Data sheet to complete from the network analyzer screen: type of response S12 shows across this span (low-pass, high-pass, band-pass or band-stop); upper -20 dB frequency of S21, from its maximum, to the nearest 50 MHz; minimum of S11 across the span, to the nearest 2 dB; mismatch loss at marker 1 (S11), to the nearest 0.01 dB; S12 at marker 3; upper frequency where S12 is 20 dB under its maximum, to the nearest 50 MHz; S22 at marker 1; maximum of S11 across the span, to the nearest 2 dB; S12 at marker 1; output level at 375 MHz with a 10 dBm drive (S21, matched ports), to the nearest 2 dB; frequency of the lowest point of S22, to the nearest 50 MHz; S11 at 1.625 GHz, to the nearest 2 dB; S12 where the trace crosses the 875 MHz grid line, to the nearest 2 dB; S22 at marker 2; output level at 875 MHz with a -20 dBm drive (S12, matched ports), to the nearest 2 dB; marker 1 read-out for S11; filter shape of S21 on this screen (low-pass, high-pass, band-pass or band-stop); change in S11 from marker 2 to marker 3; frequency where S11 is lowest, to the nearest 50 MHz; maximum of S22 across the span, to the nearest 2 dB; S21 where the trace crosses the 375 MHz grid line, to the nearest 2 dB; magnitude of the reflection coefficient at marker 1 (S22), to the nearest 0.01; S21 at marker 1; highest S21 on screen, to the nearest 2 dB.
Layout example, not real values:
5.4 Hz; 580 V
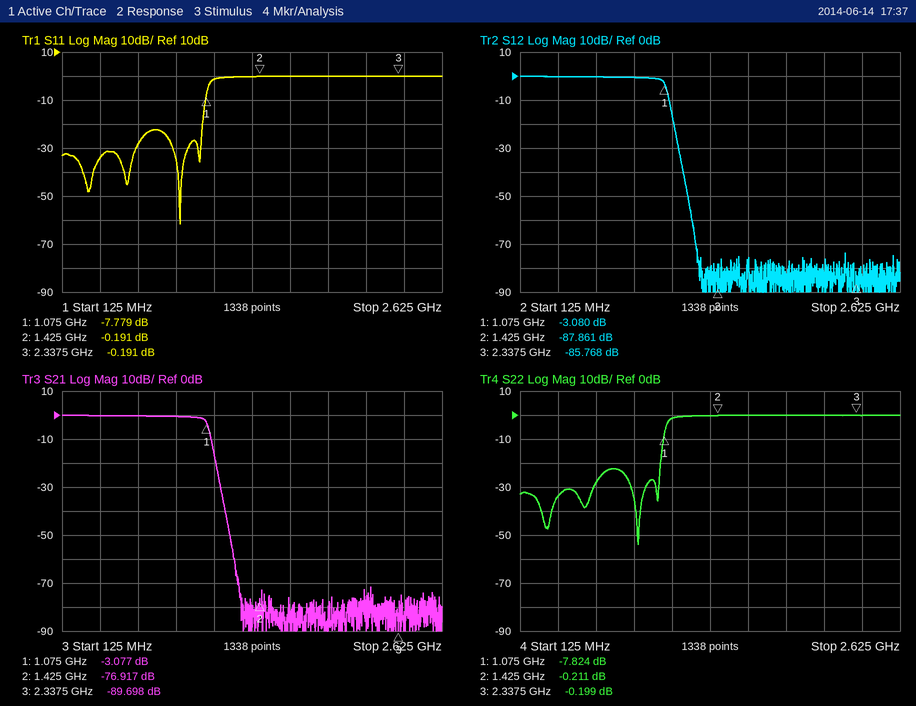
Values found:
low-pass; 1.15 GHz; -62 dB; 0.79 dB; -85.768 dB; 1.15 GHz; -7.824 dB; 0 dB; -3.080 dB; 10 dBm; 900 MHz; 0 dB; 0 dB; -0.211 dB; -20 dBm; -7.779 dB; low-pass; 0.000 dB; 900 MHz; 0 dB; 0 dB; 0.41; -3.077 dB; 0 dB
